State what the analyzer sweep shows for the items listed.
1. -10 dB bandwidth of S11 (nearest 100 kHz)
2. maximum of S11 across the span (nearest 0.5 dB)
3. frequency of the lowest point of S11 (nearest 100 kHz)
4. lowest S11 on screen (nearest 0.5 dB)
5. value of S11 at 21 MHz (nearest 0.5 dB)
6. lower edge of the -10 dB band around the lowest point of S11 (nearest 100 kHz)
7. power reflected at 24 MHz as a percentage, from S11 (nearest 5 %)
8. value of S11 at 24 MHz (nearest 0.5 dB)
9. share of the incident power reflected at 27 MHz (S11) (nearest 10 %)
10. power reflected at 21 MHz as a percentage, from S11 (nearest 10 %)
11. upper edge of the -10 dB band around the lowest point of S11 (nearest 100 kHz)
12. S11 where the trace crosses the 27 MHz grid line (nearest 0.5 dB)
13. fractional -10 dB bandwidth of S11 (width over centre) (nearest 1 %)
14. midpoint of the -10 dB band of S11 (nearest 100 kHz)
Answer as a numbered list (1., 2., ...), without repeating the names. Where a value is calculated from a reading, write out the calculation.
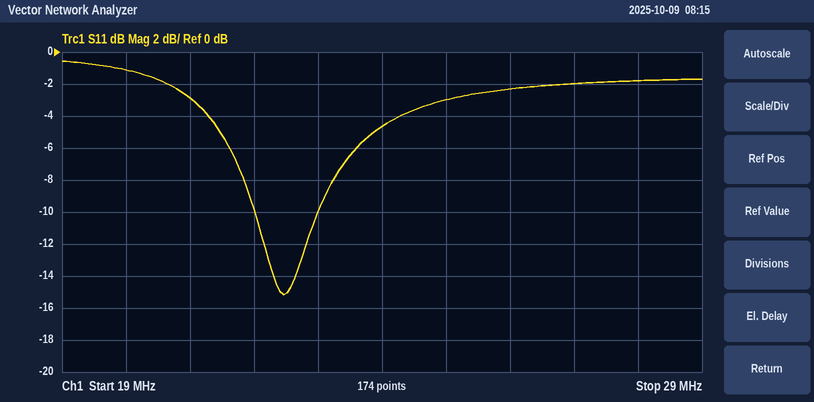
1. 23.0 MHz − 22.0 MHz = 1.0 MHz
2. -0.5 dB
3. 22.5 MHz
4. -15.0 dB
5. -3.0 dB
6. 22.0 MHz
7. 10^(-4.5/10) ≈ 35 %
8. -4.5 dB
9. 10^(-2/10) ≈ 63.1 %, so 60 % to the nearest 10 %
10. 10^(-3/10) ≈ 50 %
11. 23.0 MHz
12. -2.0 dB
13. 1 MHz / 22.5 MHz ≈ 4 %
14. 22.5 MHz
